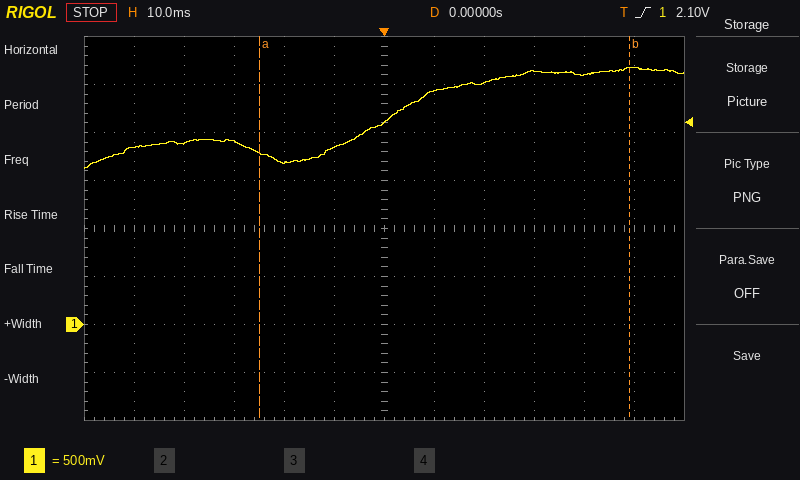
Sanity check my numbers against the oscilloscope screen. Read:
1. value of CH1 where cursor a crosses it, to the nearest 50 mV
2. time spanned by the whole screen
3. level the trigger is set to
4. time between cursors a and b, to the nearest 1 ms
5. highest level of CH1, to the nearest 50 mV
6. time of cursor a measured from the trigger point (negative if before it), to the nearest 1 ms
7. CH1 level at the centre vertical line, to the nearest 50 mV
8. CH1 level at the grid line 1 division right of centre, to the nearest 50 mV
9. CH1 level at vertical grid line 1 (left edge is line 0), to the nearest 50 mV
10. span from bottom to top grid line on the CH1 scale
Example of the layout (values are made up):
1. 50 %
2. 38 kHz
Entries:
1. 1.80 V
2. 120 ms
3. 2.10 V
4. 74 ms
5. 2.70 V
6. -25 ms
7. 2.10 V
8. 2.45 V
9. 1.85 V
10. 4 V
